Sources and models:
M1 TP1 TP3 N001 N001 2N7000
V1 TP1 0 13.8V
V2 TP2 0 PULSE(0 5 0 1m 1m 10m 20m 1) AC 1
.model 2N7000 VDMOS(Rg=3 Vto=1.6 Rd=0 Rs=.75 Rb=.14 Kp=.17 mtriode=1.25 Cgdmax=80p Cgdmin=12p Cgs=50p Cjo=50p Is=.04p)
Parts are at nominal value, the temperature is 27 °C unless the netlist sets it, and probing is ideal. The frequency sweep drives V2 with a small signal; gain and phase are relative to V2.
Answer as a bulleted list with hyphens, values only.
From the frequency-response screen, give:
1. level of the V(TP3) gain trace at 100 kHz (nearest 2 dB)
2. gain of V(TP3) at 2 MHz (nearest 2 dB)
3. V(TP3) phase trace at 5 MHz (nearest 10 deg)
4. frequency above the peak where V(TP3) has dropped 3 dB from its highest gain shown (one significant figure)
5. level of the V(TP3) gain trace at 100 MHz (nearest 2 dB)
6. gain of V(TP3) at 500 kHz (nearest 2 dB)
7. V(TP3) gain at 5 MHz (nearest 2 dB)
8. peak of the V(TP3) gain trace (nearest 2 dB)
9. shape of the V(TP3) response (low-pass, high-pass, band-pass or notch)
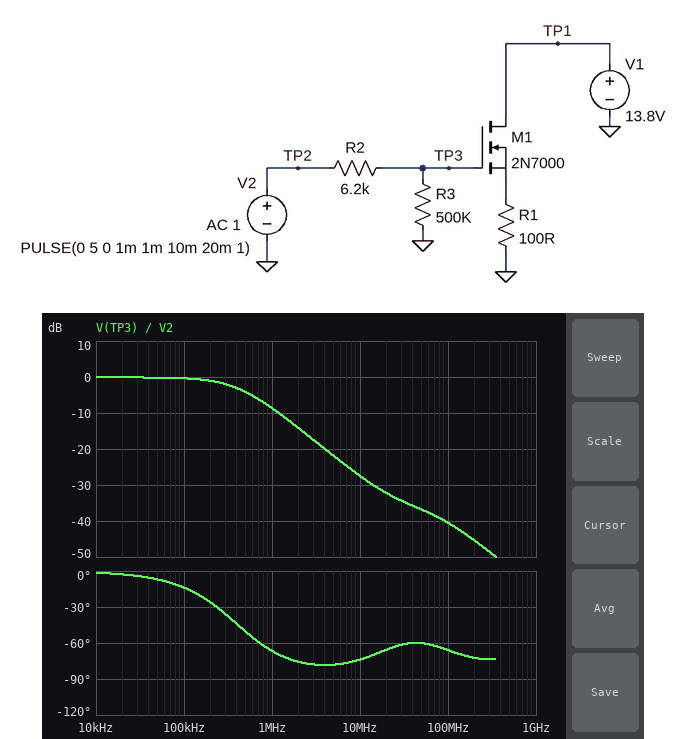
- 0 dB
- -14 dB
- -80 deg
- 400 kHz
- -40 dB
- -4 dB
- -22 dB
- 0 dB
- low-pass
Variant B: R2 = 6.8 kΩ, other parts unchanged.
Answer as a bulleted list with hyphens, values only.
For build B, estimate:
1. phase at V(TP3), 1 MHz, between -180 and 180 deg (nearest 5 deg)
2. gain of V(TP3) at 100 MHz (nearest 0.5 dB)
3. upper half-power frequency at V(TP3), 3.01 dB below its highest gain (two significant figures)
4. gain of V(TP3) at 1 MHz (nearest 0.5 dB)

- -70 deg
- -41.5 dB
- 370 kHz
- -9.5 dB
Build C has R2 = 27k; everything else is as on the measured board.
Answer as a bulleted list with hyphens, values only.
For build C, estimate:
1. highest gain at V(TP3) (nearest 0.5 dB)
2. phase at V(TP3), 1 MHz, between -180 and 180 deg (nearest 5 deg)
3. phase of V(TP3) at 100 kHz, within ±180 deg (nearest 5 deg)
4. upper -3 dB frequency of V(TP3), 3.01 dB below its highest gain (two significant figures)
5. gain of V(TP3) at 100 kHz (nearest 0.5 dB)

- -0.5 dB
- -85 deg
- -45 deg
- 97 kHz
- -3.5 dB
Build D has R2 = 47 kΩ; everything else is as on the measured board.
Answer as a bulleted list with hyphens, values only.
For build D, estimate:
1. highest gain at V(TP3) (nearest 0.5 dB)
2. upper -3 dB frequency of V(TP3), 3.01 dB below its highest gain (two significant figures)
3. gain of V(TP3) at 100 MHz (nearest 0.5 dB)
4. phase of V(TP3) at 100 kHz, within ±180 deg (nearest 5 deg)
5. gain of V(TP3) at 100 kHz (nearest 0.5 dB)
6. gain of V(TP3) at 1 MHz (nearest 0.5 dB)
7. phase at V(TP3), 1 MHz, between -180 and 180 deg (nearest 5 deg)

- -1.0 dB
- 58 kHz
- -58.0 dB
- -60 deg
- -7.0 dB
- -25.5 dB
- -85 deg
